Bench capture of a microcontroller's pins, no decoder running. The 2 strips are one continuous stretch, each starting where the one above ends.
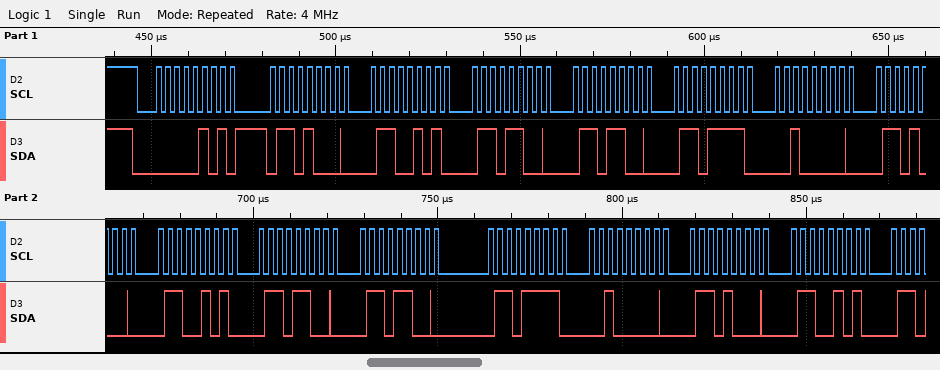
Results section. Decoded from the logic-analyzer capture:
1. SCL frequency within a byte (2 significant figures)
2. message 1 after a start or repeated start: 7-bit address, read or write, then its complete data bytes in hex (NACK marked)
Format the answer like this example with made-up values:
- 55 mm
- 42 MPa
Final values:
- 400 kHz
- 0x02 read: 68 65 6C 6C 6F 20 68 65 6C 6C 6F 20 68 65
